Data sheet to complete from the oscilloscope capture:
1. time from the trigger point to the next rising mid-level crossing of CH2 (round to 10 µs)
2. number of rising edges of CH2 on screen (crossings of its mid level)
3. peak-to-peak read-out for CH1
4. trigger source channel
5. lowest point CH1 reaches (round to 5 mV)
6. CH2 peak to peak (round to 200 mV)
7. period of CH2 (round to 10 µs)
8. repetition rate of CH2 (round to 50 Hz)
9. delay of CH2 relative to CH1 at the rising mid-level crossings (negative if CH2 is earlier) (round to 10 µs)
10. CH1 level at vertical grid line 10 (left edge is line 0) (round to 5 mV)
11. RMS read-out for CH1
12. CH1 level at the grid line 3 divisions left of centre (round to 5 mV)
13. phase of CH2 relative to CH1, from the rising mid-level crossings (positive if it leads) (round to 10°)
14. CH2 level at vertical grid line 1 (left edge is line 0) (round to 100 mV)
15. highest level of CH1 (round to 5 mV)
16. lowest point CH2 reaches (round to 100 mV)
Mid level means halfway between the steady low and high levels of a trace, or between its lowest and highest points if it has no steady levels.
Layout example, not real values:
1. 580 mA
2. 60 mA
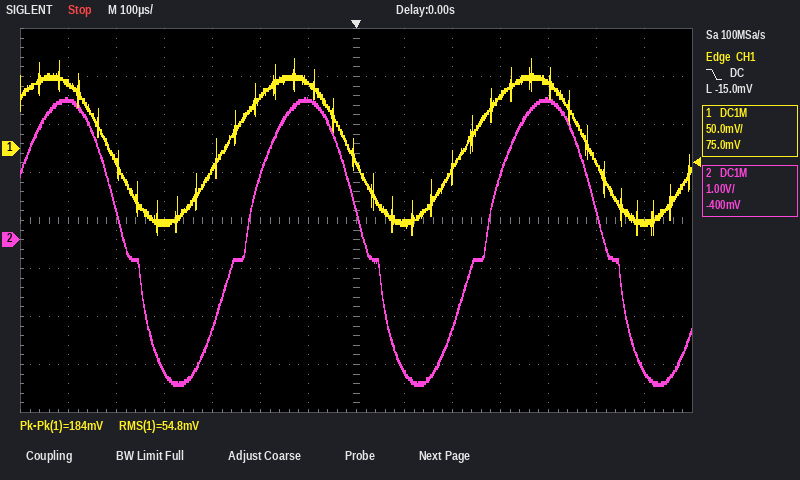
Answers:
1. 270 µs
2. 2
3. 184 mV
4. CH1
5. -90 mV
6. 6.0 V
7. 500 µs
8. 2.00 kHz
9. +40 µs
10. 55 mV
11. 54.8 mV
12. -20 mV
13. -30°
14. 2.9 V
15. 95 mV
16. -3.0 V
